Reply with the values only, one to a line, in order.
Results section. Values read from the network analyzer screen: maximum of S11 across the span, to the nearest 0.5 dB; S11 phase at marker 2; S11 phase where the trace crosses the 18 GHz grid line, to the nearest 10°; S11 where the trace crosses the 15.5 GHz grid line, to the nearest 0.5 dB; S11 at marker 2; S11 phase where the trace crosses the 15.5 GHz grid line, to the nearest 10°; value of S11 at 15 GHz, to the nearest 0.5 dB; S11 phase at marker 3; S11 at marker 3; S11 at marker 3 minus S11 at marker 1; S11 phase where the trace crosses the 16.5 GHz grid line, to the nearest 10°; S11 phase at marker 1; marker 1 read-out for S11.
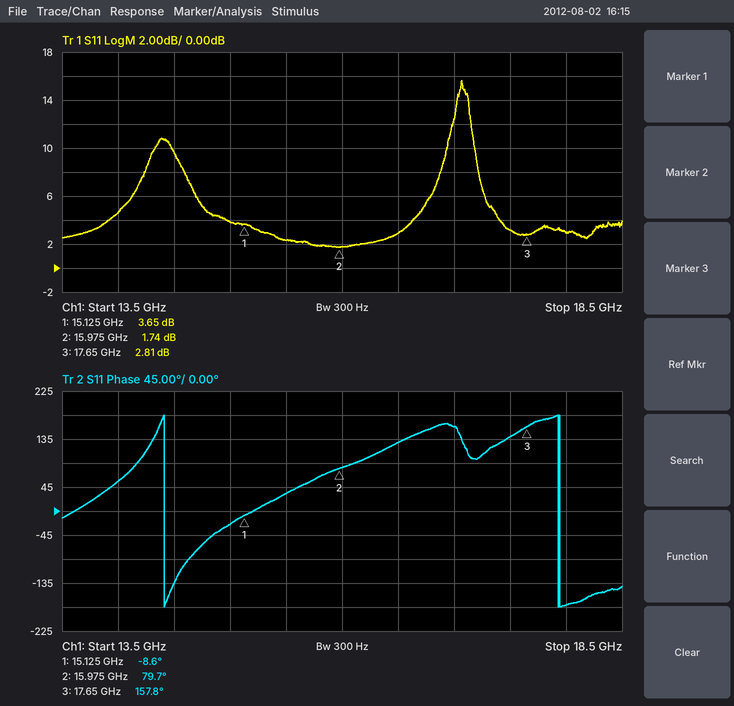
15.5 dB
79.7°
-180°
2.5 dB
1.74 dB
30°
4.0 dB
157.8°
2.81 dB
-0.84 dB
130°
-8.6°
3.65 dB
